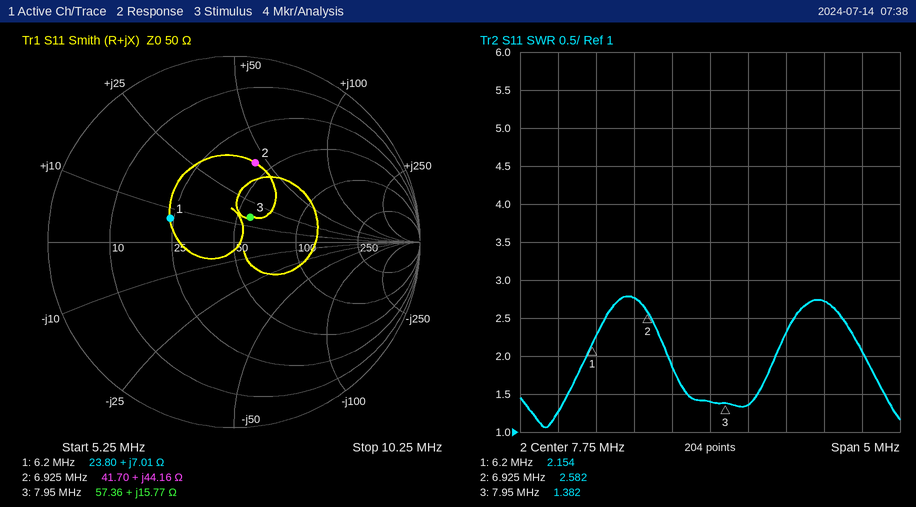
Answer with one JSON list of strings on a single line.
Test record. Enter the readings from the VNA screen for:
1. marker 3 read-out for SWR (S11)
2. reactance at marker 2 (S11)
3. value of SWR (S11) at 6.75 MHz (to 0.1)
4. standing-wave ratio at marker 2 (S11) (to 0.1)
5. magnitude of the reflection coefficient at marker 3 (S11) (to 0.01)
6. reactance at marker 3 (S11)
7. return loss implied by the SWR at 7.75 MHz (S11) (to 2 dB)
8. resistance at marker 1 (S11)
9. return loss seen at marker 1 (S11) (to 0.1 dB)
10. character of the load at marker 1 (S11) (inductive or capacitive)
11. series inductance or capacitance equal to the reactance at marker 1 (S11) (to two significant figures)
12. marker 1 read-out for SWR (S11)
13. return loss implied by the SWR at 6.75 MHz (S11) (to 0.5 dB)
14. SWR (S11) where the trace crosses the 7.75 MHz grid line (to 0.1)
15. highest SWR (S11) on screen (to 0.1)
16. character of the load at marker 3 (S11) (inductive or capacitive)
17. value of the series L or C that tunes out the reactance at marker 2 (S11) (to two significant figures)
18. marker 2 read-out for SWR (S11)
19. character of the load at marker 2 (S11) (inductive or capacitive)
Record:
["1.382", "+44.16 Ω", "2.8", "2.6", "0.16", "+15.77 Ω", "16 dB", "23.80 Ω", "8.7 dB", "inductive", "180 nH", "2.154", "6.5 dB", "1.4", "2.8", "inductive", "520 pF", "2.582", "inductive"]
